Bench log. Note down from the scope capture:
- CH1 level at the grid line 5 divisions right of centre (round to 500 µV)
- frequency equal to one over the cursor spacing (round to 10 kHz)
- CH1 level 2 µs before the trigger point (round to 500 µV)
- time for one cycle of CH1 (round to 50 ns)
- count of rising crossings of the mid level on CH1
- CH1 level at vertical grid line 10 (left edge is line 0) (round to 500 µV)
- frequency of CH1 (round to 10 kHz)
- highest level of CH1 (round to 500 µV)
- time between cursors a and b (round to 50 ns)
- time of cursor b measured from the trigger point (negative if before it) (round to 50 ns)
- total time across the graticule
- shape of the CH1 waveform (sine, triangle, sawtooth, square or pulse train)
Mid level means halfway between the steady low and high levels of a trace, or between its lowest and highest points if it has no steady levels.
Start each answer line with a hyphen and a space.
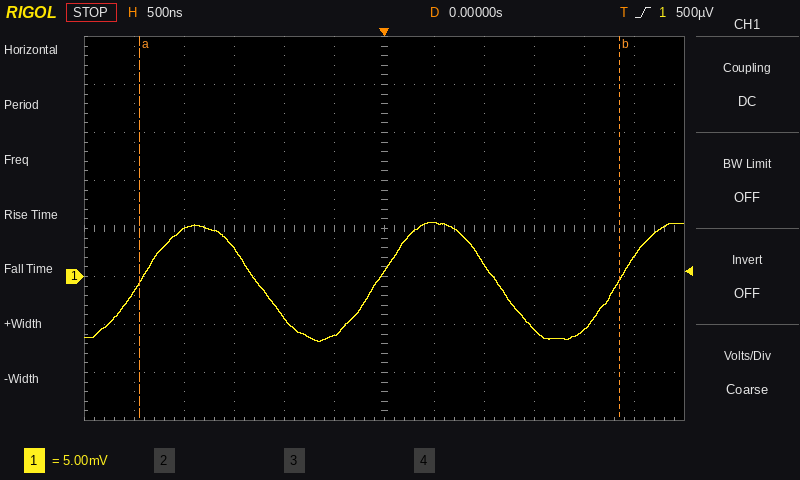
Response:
- 2.0 mV
- 210 kHz
- 5.0 mV
- 2.40 µs
- 3
- -5.5 mV
- 420 kHz
- 5.5 mV
- 4.80 µs
- +2.35 µs
- 6 µs
- sine
